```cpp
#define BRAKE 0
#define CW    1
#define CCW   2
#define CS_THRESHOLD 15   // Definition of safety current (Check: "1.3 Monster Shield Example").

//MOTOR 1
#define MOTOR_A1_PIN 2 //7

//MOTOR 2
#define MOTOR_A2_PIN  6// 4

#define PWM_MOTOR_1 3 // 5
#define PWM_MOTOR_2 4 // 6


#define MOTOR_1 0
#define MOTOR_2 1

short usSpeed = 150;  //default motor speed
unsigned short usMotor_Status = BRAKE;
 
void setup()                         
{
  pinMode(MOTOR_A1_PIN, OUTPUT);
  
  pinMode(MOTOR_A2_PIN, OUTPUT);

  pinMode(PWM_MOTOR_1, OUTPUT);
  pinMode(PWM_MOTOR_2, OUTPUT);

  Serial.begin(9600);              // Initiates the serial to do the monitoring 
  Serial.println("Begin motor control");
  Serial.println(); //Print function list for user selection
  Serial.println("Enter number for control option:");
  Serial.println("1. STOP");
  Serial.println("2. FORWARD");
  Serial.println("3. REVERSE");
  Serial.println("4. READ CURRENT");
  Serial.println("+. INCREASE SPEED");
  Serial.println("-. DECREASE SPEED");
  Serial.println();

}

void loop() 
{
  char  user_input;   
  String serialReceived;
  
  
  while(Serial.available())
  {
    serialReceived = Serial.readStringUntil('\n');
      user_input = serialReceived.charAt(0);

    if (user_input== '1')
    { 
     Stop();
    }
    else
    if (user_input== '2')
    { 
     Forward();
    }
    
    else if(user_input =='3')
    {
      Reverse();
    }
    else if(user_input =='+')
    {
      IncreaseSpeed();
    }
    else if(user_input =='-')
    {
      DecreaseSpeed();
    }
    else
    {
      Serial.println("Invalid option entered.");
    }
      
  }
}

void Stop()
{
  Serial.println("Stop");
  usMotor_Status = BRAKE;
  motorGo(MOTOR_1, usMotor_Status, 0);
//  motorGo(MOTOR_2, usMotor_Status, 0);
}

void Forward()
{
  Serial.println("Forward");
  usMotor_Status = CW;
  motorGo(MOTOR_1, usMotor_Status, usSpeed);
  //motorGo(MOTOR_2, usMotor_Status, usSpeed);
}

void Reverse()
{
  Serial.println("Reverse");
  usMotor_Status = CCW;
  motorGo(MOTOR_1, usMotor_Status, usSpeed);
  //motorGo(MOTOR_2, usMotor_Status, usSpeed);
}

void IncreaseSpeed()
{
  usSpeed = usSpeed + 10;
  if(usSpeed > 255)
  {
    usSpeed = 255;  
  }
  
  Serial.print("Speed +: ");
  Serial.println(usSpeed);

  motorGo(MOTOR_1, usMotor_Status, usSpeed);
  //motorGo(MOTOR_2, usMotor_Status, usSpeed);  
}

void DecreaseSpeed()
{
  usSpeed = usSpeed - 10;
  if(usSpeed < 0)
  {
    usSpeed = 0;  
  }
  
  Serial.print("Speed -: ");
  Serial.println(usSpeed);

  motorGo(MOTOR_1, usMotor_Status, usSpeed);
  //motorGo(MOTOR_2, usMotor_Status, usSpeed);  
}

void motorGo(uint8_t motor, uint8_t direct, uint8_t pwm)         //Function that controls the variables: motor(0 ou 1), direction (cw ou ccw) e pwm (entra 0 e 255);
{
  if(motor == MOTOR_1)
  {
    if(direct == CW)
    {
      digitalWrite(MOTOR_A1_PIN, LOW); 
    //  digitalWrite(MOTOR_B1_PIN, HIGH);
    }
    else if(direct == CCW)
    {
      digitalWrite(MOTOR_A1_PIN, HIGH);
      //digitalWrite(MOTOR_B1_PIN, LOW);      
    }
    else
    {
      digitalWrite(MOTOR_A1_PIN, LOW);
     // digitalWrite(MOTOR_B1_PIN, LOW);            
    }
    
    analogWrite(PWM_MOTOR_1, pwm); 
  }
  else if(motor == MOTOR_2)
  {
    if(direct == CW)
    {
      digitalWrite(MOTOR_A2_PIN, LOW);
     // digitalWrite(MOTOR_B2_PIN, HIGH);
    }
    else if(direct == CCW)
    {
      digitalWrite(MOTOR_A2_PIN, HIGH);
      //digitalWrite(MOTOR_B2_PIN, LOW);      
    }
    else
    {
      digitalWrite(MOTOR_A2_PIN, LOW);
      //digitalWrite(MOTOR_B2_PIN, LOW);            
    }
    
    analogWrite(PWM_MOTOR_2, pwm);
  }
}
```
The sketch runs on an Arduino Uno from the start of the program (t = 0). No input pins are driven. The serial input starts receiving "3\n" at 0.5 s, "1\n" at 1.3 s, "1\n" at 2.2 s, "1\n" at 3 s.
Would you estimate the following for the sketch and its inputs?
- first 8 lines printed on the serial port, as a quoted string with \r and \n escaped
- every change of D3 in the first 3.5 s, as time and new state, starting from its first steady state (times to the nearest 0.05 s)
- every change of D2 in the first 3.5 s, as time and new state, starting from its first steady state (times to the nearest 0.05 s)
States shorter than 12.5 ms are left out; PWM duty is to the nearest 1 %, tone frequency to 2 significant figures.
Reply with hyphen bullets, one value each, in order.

- "Begin motor control\r\n\r\nEnter number for control option:\r\n1. STOP\r\n2. FORWARD\r\n3. REVERSE\r\n4. READ CURRENT\r\n+. INCREASE SPEED\r\n"
- 0 s low; 0.5 s PWM 59 %; 1.3 s low
- 0 s low; 0.5 s high; 1.3 s low
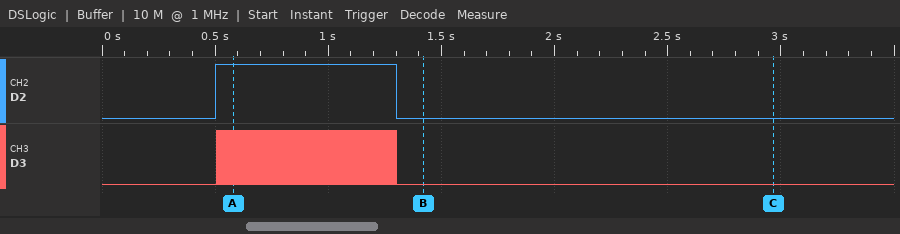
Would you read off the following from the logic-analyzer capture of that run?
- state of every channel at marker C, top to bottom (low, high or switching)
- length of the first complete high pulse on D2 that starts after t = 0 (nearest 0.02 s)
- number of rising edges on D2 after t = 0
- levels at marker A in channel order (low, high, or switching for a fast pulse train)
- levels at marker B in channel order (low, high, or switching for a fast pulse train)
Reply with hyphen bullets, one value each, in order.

- D2 low, D3 low
- 0.80 s
- 1
- D2 high, D3 switching
- D2 low, D3 low
